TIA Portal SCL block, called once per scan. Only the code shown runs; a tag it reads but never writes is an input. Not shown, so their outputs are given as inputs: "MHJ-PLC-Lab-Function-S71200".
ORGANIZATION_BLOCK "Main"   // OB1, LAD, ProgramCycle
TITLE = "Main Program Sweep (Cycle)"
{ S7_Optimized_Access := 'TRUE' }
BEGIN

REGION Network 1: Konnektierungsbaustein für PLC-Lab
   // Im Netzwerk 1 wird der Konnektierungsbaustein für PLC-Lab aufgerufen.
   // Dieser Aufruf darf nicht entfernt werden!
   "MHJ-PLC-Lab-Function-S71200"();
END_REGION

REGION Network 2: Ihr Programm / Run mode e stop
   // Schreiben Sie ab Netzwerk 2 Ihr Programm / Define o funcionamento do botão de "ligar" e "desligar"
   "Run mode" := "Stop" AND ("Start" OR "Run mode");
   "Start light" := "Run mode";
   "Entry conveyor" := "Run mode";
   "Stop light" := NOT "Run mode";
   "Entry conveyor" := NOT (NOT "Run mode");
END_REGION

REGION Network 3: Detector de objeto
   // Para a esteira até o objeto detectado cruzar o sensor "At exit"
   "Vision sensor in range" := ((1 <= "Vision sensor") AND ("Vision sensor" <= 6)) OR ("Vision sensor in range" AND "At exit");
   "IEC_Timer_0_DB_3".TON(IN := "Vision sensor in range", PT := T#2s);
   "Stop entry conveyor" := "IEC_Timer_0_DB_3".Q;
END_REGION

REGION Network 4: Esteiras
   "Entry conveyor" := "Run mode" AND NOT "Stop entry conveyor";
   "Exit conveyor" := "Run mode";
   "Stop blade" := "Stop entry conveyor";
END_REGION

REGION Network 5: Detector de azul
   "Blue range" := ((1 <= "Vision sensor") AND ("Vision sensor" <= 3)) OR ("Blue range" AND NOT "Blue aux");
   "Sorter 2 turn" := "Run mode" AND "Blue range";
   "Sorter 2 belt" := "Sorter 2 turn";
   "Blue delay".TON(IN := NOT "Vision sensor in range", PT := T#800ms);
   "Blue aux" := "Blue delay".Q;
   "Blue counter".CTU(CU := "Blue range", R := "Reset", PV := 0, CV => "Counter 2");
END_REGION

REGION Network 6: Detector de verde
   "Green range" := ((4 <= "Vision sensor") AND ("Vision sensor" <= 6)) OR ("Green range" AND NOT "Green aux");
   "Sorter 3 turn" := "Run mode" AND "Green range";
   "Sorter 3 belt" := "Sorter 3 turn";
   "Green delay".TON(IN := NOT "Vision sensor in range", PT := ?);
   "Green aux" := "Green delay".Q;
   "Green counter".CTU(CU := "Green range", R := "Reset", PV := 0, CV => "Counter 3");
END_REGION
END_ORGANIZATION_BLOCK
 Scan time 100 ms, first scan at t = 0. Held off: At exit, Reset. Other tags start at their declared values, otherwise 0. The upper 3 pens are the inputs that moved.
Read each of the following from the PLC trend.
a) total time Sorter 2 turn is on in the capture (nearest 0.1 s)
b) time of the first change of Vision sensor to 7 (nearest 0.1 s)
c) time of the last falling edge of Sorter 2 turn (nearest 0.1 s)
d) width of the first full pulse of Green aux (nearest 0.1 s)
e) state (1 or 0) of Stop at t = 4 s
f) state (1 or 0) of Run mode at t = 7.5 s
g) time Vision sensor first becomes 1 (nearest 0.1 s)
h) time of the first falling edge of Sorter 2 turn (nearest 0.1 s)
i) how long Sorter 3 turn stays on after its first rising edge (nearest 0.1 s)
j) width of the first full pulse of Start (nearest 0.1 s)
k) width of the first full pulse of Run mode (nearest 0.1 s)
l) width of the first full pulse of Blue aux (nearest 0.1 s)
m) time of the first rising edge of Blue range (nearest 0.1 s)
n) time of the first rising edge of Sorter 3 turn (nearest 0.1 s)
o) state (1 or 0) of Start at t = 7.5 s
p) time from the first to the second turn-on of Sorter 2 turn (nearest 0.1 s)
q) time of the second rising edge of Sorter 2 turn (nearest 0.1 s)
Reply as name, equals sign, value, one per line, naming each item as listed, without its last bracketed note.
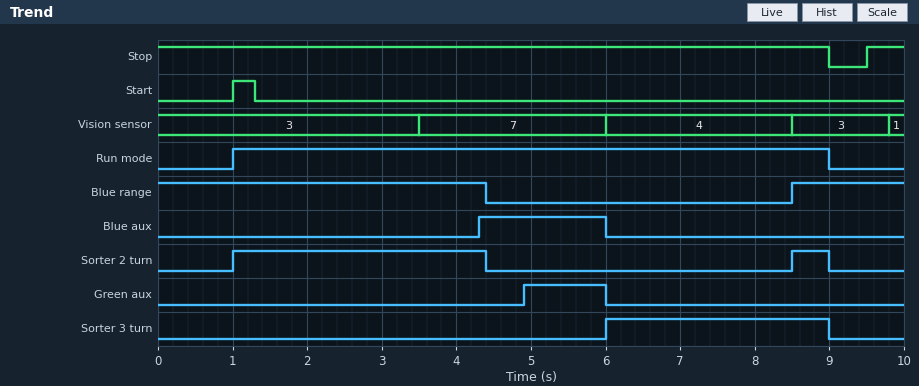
total time Sorter 2 turn is on in the capture = 3.9 s
time of the first change of Vision sensor to 7 = 3.5 s
time of the last falling edge of Sorter 2 turn = 9.0 s
width of the first full pulse of Green aux = 1.1 s
state (1 or 0) of Stop at t = 4 s = 1
state (1 or 0) of Run mode at t = 7.5 s = 1
time Vision sensor first becomes 1 = 9.8 s
time of the first falling edge of Sorter 2 turn = 4.4 s
how long Sorter 3 turn stays on after its first rising edge = 3.0 s
width of the first full pulse of Start = 0.3 s
width of the first full pulse of Run mode = 8.0 s
width of the first full pulse of Blue aux = 1.7 s
time of the first rising edge of Blue range = 8.5 s
time of the first rising edge of Sorter 3 turn = 6.0 s
state (1 or 0) of Start at t = 7.5 s = 0
time from the first to the second turn-on of Sorter 2 turn = 7.5 s
time of the second rising edge of Sorter 2 turn = 8.5 s
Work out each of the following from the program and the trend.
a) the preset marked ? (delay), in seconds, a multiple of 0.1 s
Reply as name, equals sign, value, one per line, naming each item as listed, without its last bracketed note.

the preset marked ? (delay), in seconds, a multiple of 0.1 s = 1.4 s
